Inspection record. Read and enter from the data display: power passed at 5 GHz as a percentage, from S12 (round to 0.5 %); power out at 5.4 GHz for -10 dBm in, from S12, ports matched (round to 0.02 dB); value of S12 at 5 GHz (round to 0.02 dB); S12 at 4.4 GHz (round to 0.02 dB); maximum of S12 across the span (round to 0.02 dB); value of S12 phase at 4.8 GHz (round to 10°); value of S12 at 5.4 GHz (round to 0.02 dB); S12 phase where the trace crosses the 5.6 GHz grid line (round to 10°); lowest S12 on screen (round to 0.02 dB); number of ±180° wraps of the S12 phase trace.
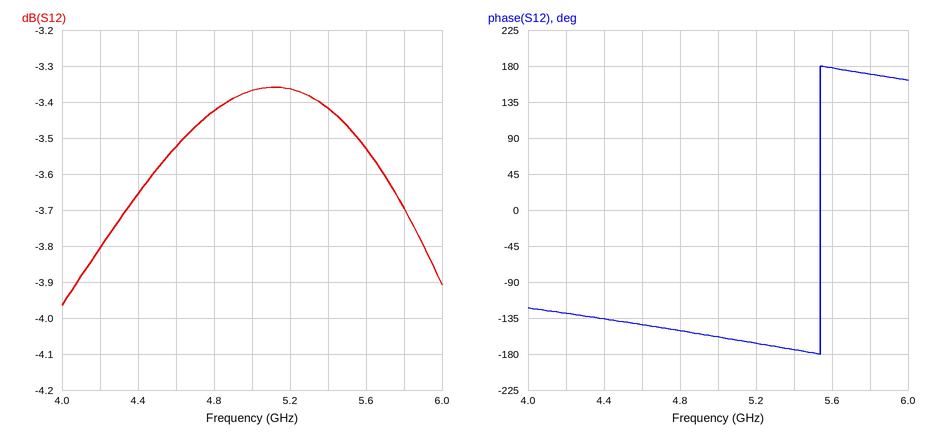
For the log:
46.0 %
-13.42 dBm
-3.36 dB
-3.66 dB
-3.36 dB
-150°
-3.42 dB
180°
-3.96 dB
1
